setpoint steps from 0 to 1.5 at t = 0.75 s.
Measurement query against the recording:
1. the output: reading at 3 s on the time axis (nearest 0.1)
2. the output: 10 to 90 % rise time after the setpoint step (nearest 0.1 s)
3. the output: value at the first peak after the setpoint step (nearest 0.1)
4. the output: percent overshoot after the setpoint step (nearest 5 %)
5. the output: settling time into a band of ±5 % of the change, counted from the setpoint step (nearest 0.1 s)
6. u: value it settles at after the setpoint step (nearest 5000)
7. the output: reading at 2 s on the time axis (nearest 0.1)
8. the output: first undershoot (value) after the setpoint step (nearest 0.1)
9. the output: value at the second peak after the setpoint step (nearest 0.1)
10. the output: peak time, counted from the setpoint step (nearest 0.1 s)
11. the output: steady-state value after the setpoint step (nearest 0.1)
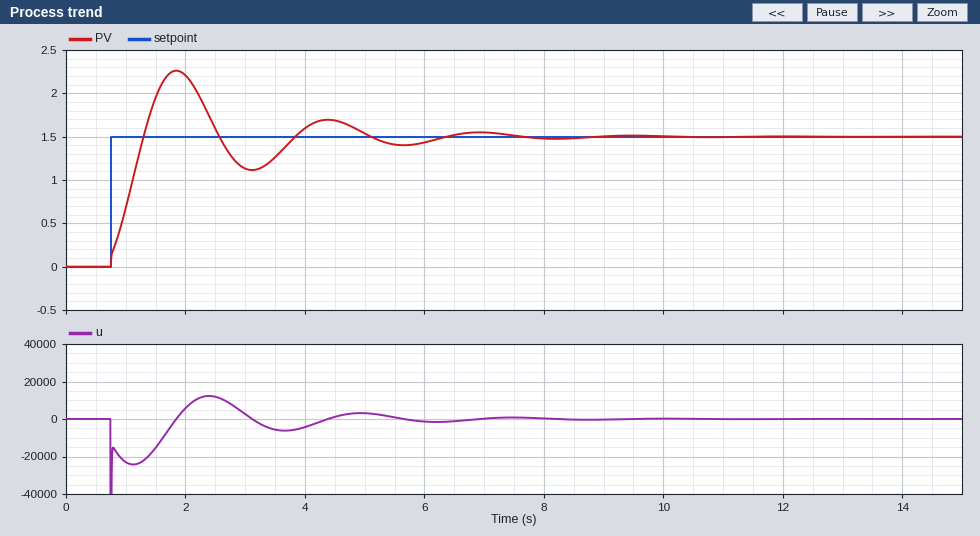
1.1
0.5 s
2.3
50 %
5.2 s
0
2.2
1.1
1.7
1.1 s
1.5
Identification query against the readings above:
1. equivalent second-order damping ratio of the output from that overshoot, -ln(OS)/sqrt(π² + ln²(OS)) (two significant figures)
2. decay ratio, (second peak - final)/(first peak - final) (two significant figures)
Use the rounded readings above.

0.22
0.25
